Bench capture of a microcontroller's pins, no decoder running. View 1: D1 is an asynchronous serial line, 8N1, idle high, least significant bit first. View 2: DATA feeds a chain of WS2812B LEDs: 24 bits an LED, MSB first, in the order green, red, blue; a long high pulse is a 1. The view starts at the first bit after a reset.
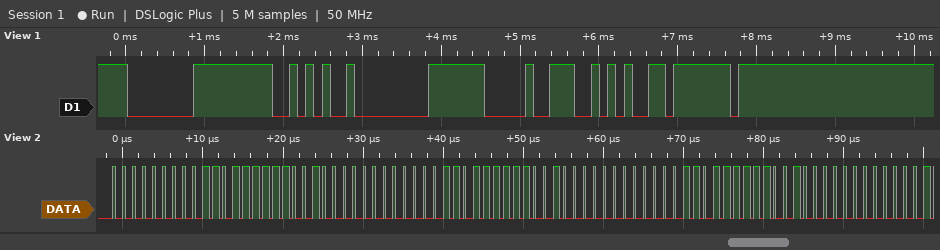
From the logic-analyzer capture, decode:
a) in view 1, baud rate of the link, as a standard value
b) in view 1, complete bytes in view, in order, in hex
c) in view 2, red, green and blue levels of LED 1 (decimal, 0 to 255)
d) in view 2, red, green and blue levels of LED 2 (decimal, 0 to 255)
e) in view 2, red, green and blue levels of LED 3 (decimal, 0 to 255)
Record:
9600 baud
80 2A 00 90 2A 7F
111, 0, 200
111, 0, 200
111, 0, 200
